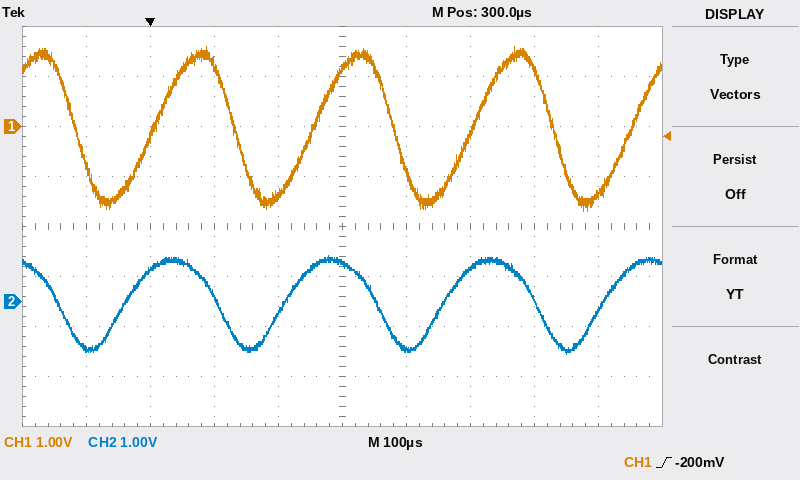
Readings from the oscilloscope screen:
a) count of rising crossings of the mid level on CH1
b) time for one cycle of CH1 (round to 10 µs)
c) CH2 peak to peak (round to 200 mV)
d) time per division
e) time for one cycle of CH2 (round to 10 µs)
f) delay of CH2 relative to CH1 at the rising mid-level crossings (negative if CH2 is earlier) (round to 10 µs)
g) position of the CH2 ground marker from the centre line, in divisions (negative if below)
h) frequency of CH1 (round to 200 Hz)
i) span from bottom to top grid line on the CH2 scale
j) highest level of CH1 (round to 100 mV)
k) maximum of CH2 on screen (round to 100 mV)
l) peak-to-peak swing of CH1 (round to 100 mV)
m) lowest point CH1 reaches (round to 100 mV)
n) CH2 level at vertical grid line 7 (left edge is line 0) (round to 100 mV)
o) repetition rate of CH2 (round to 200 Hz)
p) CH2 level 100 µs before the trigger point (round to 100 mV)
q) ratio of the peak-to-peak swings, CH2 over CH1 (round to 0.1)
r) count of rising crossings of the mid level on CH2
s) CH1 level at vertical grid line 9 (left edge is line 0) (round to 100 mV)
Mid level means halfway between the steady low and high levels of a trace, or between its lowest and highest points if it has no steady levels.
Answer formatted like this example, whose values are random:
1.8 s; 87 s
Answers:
4; 250 µs; 2.0 V; 100 µs; 250 µs; -50 µs; -1.5 div; 4.0 kHz; 8 V; 1.6 V; 900 mV; 3.3 V; -1.7 V; 700 mV; 4.0 kHz; -900 mV; 0.6; 4; -1.3 V
